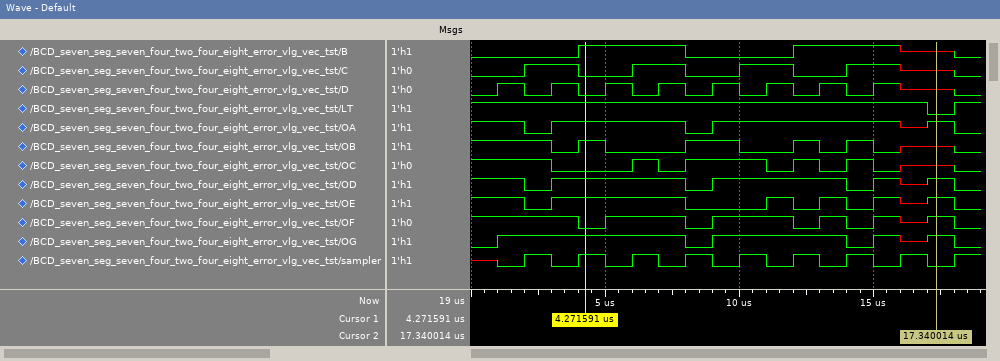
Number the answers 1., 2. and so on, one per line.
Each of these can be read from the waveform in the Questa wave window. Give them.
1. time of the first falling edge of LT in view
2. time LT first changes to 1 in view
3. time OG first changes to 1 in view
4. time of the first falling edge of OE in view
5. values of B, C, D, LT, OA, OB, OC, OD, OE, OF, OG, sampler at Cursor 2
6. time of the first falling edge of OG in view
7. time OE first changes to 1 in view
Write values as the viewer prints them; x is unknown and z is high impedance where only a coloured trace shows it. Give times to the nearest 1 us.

1. 17 us
2. 18 us
3. 1 us
4. 2 us
5. B=x, C=x, D=x, LT=0, OA=1, OB=x, OC=x, OD=1, OE=1, OF=1, OG=1, sampler=0
6. 8 us
7. 3 us
